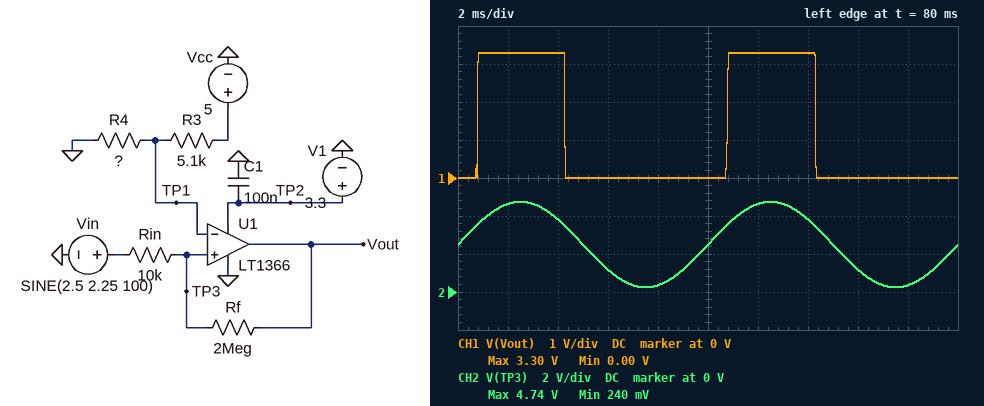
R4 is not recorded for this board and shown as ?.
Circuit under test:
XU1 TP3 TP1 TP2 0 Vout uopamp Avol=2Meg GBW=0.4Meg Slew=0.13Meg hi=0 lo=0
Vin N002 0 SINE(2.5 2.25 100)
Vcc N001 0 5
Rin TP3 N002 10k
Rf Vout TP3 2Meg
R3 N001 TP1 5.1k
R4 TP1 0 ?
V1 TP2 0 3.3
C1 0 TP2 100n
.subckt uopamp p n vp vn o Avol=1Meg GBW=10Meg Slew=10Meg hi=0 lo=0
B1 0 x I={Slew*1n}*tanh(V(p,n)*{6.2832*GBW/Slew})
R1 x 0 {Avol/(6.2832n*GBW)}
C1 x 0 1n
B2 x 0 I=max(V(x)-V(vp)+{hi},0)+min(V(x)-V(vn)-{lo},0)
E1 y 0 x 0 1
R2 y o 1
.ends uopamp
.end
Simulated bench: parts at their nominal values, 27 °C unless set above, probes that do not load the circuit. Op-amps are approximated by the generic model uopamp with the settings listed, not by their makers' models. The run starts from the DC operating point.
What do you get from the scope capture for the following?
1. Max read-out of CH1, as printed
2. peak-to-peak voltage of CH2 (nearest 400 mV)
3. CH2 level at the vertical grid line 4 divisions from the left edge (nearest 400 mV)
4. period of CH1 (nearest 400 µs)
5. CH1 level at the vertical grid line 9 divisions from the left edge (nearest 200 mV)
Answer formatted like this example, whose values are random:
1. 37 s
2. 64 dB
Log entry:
1. 3.30 V
2. 4.4 V
3. 400 mV
4. 10.0 ms
5. 0 V
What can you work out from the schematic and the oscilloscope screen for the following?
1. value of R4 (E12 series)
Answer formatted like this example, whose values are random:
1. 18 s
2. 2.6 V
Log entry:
1. 12 kΩ
